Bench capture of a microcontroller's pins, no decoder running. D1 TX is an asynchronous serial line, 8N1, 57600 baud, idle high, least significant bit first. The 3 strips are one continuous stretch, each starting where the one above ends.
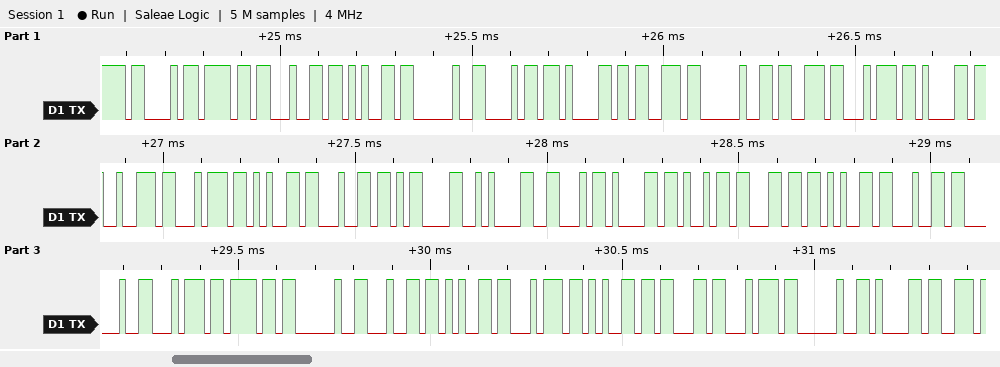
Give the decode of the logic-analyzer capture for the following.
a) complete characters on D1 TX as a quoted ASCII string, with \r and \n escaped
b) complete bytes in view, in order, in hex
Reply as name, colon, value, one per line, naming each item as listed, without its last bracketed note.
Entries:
complete characters on D1 TX as a quoted ASCII string, with \r and \n escaped: "Code has started\r\nFailed to detect a"
complete bytes in view, in order, in hex: 43 6F 64 65 20 68 61 73 20 73 74 61 72 74 65 64 0D 0A 46 61 69 6C 65 64 20 74 6F 20 64 65 74 65 63 74 20 61
